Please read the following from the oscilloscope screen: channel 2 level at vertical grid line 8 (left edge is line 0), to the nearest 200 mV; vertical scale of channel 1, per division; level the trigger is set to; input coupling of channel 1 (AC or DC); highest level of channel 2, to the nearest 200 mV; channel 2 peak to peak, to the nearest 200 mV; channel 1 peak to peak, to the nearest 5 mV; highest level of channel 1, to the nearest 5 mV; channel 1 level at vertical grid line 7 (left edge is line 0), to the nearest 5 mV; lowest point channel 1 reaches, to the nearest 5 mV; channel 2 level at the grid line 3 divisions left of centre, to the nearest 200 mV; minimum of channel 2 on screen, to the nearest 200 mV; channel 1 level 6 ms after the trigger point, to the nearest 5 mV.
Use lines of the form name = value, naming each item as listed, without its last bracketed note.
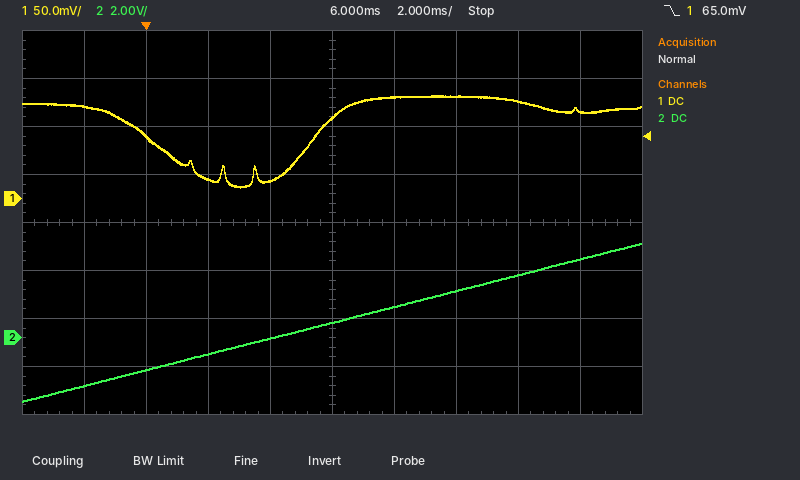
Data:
channel 2 level at vertical grid line 8 (left edge is line 0), to the nearest 200 mV = 2.6 V
vertical scale of channel 1, per division = 50 mV
level the trigger is set to = 65.0 mV
input coupling of channel 1 = DC
highest level of channel 2, to the nearest 200 mV = 4.0 V
channel 2 peak to peak, to the nearest 200 mV = 6.6 V
channel 1 peak to peak, to the nearest 5 mV = 95 mV
highest level of channel 1, to the nearest 5 mV = 105 mV
channel 1 level at vertical grid line 7 (left edge is line 0), to the nearest 5 mV = 105 mV
lowest point channel 1 reaches, to the nearest 5 mV = 10 mV
channel 2 level at the grid line 3 divisions left of centre, to the nearest 200 mV = -1.4 V
minimum of channel 2 on screen, to the nearest 200 mV = -2.6 V
channel 1 level 6 ms after the trigger point, to the nearest 5 mV = 85 mV
